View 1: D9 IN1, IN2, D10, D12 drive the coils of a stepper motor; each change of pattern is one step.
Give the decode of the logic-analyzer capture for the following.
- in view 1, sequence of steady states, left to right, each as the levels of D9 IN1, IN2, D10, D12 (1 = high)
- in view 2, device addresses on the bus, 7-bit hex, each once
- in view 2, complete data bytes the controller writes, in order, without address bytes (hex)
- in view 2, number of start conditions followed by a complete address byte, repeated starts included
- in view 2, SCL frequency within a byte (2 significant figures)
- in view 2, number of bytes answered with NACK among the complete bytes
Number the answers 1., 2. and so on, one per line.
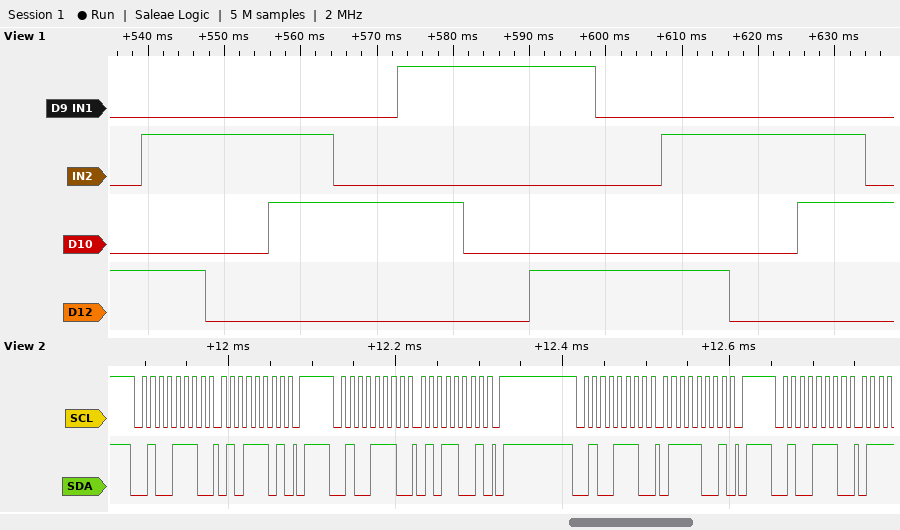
1. 0001 0101 0100 0110 0010 1010 1000 1001 0001 0101 0100 0110 0010
2. 0x27
3. 5D 59 79
4. 4
5. 100 kHz
6. 0
